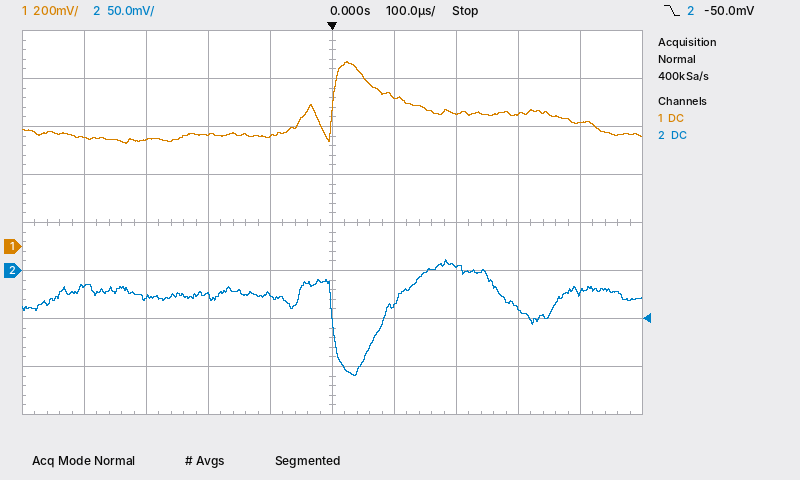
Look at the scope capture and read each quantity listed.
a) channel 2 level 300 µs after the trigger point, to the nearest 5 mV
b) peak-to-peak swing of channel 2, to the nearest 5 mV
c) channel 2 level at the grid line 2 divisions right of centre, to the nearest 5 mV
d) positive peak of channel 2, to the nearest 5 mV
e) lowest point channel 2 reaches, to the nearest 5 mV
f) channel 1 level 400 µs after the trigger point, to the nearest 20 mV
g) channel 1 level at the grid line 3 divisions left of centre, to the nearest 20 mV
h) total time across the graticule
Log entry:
-40 mV
120 mV
5 mV
10 mV
-110 mV
520 mV
440 mV
1 ms
